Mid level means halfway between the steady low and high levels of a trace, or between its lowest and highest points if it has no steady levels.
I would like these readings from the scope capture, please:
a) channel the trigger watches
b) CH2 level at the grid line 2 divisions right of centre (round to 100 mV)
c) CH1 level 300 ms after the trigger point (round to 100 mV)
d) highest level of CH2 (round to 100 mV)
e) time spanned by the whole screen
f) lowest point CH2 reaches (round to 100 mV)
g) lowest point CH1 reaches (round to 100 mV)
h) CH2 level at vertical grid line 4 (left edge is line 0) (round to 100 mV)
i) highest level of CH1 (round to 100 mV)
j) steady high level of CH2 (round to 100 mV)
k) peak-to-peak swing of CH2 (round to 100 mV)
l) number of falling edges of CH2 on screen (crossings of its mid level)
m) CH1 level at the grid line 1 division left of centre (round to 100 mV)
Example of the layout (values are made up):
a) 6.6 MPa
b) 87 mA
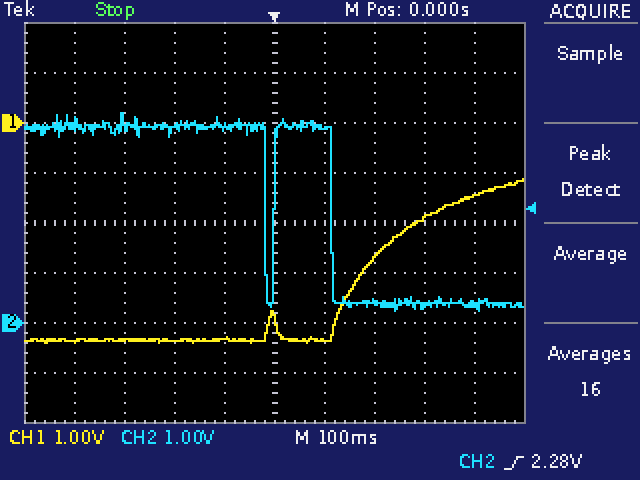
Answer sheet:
a) CH2
b) 400 mV
c) -1.9 V
d) 4.2 V
e) 1 s
f) 200 mV
g) -4.4 V
h) 3.9 V
i) -1.1 V
j) 3.9 V
k) 4.0 V
l) 2
m) -4.3 V
